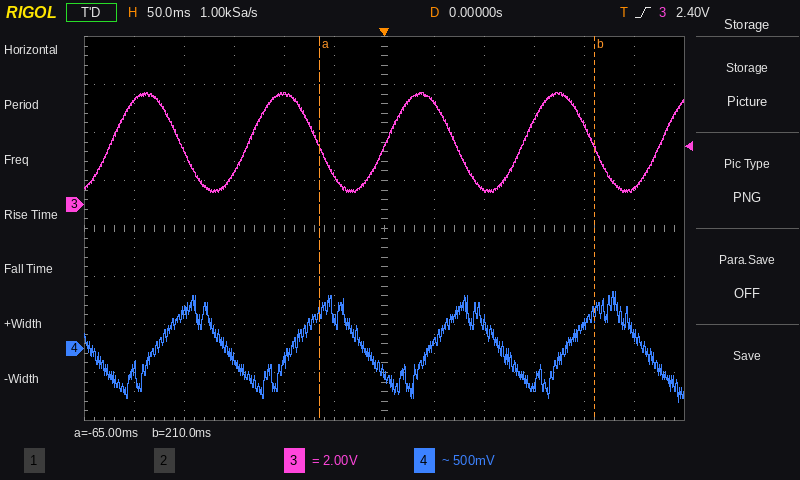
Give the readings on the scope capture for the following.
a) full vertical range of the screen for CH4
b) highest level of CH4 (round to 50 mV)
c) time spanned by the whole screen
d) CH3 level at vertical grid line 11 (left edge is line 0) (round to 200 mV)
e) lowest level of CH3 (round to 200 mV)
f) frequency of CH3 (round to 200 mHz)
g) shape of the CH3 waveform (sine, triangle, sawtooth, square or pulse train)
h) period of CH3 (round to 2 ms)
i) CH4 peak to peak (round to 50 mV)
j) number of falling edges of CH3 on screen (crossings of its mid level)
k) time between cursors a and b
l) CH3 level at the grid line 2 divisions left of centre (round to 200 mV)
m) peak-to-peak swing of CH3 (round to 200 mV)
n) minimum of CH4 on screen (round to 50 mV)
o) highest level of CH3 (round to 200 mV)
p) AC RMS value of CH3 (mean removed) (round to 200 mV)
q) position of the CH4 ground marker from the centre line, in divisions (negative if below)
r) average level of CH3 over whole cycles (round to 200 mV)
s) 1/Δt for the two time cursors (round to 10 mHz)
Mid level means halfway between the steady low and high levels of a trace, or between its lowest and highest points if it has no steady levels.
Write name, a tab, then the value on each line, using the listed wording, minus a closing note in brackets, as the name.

full vertical range of the screen for CH4	4 V
highest level of CH4	600 mV
time spanned by the whole screen	600 ms
CH3 level at vertical grid line 11 (left edge is line 0)	600 mV
lowest level of CH3	400 mV
frequency of CH3	7.2 Hz
shape of the CH3 waveform	sine
period of CH3	138 ms
CH4 peak to peak	1.15 V
number of falling edges of CH3 on screen	4
time between cursors a and b	275 ms
CH3 level at the grid line 2 divisions left of centre	4.6 V
peak-to-peak swing of CH3	4.2 V
minimum of CH4 on screen	-550 mV
highest level of CH3	4.6 V
AC RMS value of CH3 (mean removed)	1.4 V
position of the CH4 ground marker from the centre line, in divisions	-2.5 div
average level of CH3 over whole cycles	2.6 V
1/Δt for the two time cursors	3.64 Hz
